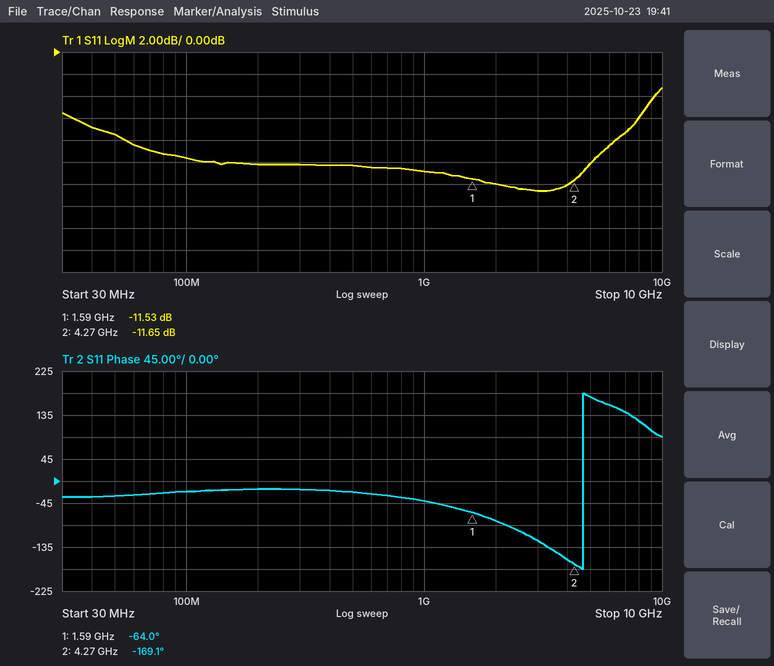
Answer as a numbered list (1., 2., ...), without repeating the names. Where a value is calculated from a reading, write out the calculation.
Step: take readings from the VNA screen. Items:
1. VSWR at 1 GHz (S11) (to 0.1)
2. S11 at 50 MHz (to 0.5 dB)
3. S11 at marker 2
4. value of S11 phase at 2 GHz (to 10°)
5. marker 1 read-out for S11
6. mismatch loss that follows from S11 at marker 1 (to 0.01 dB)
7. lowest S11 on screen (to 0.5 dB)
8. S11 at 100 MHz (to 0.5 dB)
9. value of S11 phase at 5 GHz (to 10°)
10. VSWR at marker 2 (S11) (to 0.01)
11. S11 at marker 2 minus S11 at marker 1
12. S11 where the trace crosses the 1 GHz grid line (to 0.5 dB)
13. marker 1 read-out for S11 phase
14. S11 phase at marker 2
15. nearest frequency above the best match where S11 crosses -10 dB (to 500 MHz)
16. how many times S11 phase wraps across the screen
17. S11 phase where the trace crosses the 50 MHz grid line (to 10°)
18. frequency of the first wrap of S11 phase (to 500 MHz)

1. |Γ| = 10^(-11/20) = 0.2818; VSWR = (1 + 0.2818)/(1 − 0.2818) ≈ 1.8
2. -7.5 dB
3. -11.65 dB
4. -80°
5. -11.53 dB
6. −10 log10(1 − 10^(-11.53/10)) ≈ 0.32 dB
7. -12.5 dB
8. -9.5 dB
9. 170°
10. (1 + 0.2615)/(1 − 0.2615) ≈ 1.71
11. -11.65 − (-11.53) = -0.12 dB
12. -11.0 dB
13. -64.0°
14. -169.1°
15. 5.0 GHz
16. 1
17. -30°
18. 4.5 GHz
